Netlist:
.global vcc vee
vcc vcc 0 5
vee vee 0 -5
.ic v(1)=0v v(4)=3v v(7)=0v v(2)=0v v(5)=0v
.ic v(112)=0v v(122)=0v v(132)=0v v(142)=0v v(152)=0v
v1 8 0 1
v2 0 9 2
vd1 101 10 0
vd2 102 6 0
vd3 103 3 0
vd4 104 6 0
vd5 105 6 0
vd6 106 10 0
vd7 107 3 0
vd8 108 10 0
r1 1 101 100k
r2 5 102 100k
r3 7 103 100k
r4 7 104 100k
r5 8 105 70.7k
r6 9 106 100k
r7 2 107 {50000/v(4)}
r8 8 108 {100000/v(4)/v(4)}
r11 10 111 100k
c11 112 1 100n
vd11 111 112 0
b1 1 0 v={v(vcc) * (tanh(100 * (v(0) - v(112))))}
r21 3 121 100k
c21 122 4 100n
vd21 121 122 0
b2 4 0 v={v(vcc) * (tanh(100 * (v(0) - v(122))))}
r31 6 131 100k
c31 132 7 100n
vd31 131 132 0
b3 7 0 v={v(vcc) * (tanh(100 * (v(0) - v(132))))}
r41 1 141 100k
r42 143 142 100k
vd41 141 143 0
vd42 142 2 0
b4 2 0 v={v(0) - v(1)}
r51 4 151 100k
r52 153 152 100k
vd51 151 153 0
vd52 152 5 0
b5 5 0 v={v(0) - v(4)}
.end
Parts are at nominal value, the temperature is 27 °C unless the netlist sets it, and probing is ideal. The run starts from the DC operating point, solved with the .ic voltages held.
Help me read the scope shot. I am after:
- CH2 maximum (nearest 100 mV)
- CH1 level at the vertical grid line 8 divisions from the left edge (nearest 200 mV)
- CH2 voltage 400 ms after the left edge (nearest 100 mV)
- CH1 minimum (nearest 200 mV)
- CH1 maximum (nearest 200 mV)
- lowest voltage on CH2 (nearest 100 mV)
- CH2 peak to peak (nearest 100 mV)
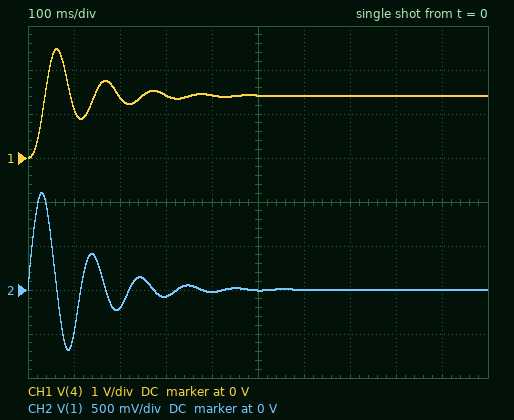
1.1 V
1.4 V
0 V
0 V
2.4 V
-700 mV
1.8 V
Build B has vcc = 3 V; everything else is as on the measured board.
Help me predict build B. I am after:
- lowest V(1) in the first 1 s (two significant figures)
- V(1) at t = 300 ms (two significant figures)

-670 mV
-70 mV
